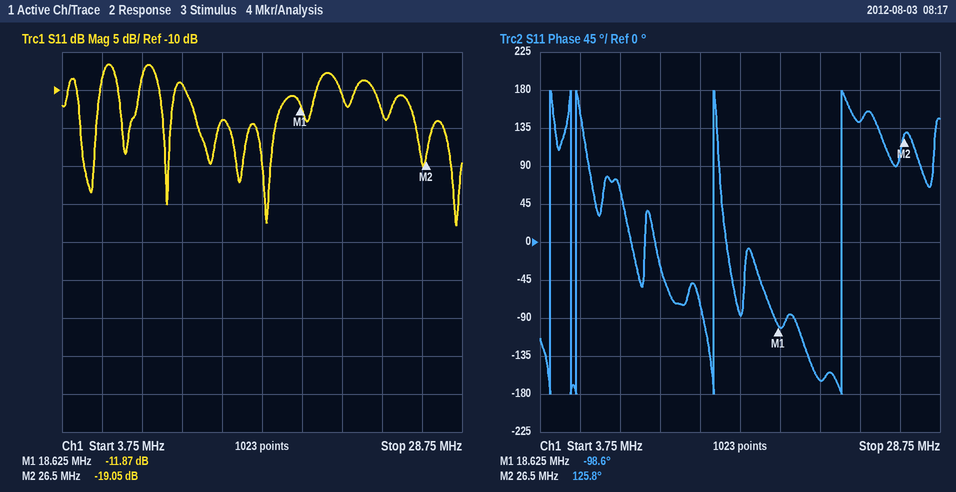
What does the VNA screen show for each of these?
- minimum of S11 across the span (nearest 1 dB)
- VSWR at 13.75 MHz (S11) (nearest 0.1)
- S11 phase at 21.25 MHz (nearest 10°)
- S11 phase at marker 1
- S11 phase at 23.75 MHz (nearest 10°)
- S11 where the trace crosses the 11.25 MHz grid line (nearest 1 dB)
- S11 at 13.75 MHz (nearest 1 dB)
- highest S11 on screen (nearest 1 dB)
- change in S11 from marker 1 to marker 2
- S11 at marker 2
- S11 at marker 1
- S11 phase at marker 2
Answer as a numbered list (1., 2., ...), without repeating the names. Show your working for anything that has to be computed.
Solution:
1. -28 dB
2. |Γ| = 10^(-14/20) = 0.1995; VSWR = (1 + 0.1995)/(1 − 0.1995) ≈ 1.5
3. -160°
4. -98.6°
5. 140°
6. -9 dB
7. -14 dB
8. -7 dB
9. -19.05 − (-11.87) = -7.18 dB
10. -19.05 dB
11. -11.87 dB
12. 125.8°
